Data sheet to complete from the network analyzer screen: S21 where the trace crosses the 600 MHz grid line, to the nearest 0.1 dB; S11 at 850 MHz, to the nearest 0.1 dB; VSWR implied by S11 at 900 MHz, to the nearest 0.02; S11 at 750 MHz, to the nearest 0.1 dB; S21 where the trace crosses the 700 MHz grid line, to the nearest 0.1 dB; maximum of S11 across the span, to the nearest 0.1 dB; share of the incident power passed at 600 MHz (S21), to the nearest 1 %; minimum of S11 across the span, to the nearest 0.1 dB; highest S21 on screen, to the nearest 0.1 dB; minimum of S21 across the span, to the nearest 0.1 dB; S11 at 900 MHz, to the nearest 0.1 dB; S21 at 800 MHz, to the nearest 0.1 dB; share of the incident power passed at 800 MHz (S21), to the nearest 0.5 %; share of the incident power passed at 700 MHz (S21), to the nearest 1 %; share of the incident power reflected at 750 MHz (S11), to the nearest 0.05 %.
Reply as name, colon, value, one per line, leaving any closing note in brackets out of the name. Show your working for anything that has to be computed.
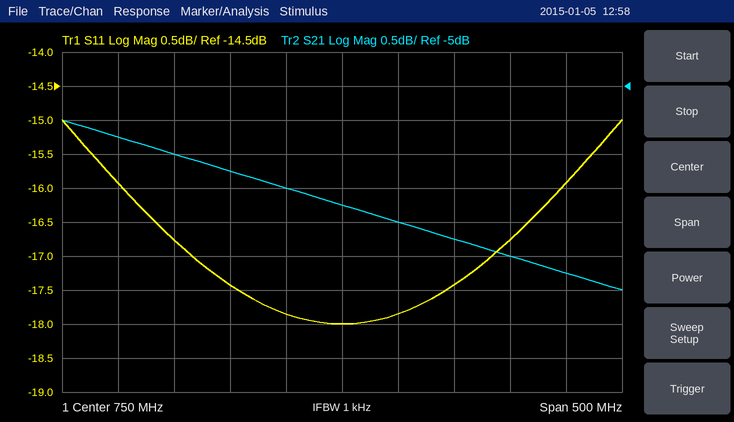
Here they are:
S21 where the trace crosses the 600 MHz grid line, to the nearest 0.1 dB: -6.0 dB
S11 at 850 MHz, to the nearest 0.1 dB: -17.4 dB
VSWR implied by S11 at 900 MHz, to the nearest 0.02: |Γ| = 10^(-16.8/20) = 0.1445; VSWR = (1 + 0.1445)/(1 − 0.1445) ≈ 1.34
S11 at 750 MHz, to the nearest 0.1 dB: -18.0 dB
S21 where the trace crosses the 700 MHz grid line, to the nearest 0.1 dB: -6.5 dB
maximum of S11 across the span, to the nearest 0.1 dB: -15.0 dB
share of the incident power passed at 600 MHz (S21), to the nearest 1 %: 10^(-6/10) ≈ 25 %
minimum of S11 across the span, to the nearest 0.1 dB: -18.0 dB
highest S21 on screen, to the nearest 0.1 dB: -5.5 dB
minimum of S21 across the span, to the nearest 0.1 dB: -8.0 dB
S11 at 900 MHz, to the nearest 0.1 dB: -16.8 dB
S21 at 800 MHz, to the nearest 0.1 dB: -7.0 dB
share of the incident power passed at 800 MHz (S21), to the nearest 0.5 %: 10^(-7/10) ≈ 20.0 %
share of the incident power passed at 700 MHz (S21), to the nearest 1 %: 10^(-6.5/10) ≈ 22 %
share of the incident power reflected at 750 MHz (S11), to the nearest 0.05 %: 10^(-18/10) ≈ 1.58 %, so 1.60 % to the nearest 0.05 %
